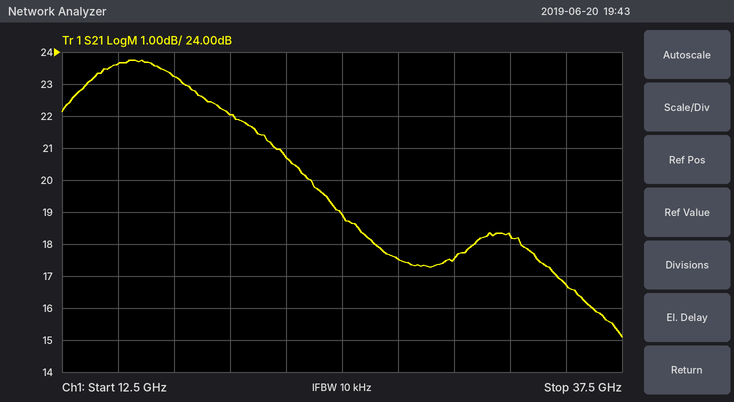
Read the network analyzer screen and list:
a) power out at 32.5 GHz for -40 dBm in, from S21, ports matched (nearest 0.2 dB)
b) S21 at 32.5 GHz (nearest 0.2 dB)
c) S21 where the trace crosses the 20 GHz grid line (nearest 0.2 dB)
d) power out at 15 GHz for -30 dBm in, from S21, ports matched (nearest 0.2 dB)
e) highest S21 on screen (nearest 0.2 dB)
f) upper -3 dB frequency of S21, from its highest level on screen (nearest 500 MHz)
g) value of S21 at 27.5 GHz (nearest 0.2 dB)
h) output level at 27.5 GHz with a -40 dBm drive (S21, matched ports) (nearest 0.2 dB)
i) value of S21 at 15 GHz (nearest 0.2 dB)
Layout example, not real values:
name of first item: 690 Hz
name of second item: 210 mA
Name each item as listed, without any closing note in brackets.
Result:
power out at 32.5 GHz for -40 dBm in, from S21, ports matched: -21.8 dBm
S21 at 32.5 GHz: 18.2 dB
S21 where the trace crosses the 20 GHz grid line: 22.0 dB
power out at 15 GHz for -30 dBm in, from S21, ports matched: -6.4 dBm
highest S21 on screen: 23.8 dB
upper -3 dB frequency of S21, from its highest level on screen: 22.5 GHz
value of S21 at 27.5 GHz: 17.6 dB
output level at 27.5 GHz with a -40 dBm drive (S21, matched ports): -22.4 dBm
value of S21 at 15 GHz: 23.6 dB
